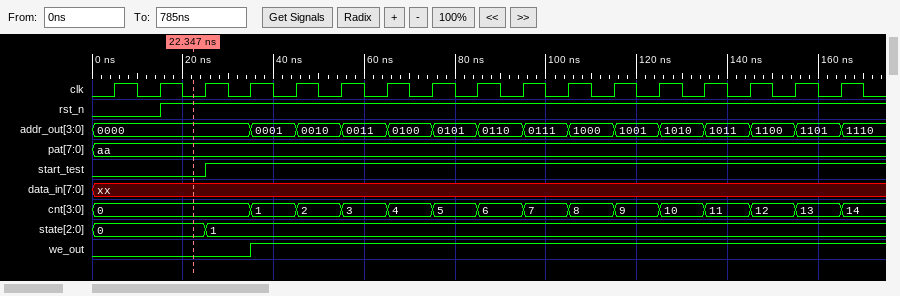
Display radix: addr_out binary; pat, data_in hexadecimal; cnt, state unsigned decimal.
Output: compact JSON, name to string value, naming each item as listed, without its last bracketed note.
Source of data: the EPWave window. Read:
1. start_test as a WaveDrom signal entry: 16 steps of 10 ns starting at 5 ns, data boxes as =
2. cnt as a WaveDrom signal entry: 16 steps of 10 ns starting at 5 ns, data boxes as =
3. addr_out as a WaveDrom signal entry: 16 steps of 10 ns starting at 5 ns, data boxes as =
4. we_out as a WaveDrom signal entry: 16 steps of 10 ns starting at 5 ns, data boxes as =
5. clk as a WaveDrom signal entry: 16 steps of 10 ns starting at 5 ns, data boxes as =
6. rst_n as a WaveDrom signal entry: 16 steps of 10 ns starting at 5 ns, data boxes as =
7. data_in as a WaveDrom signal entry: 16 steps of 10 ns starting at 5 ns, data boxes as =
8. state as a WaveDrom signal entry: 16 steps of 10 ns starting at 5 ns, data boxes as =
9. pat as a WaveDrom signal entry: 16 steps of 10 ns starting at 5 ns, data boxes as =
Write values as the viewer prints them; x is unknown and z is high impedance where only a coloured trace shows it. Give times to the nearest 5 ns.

{"start_test as a WaveDrom signal entry: 16 steps of 10 ns starting at 5 ns, data boxes as =": "{name: 'start_test', wave: '0.1.............'}", "cnt as a WaveDrom signal entry: 16 steps of 10 ns starting at 5 ns, data boxes as =": "{name: 'cnt', wave: '=..=============', data: '0 1 2 3 4 5 6 7 8 9 10 11 12 13'}", "addr_out as a WaveDrom signal entry: 16 steps of 10 ns starting at 5 ns, data boxes as =": "{name: 'addr_out', wave: '=..=============', data: '0000 0001 0010 0011 0100 0101 0110 0111 1000 1001 1010 1011 1100 1101'}", "we_out as a WaveDrom signal entry: 16 steps of 10 ns starting at 5 ns, data boxes as =": "{name: 'we_out', wave: '0..1............'}", "clk as a WaveDrom signal entry: 16 steps of 10 ns starting at 5 ns, data boxes as =": "{name: 'clk', wave: 'p...............'}", "rst_n as a WaveDrom signal entry: 16 steps of 10 ns starting at 5 ns, data boxes as =": "{name: 'rst_n', wave: '01..............'}", "data_in as a WaveDrom signal entry: 16 steps of 10 ns starting at 5 ns, data boxes as =": "{name: 'data_in', wave: 'x...............'}", "state as a WaveDrom signal entry: 16 steps of 10 ns starting at 5 ns, data boxes as =": "{name: 'state', wave: '=.=.............', data: '0 1'}", "pat as a WaveDrom signal entry: 16 steps of 10 ns starting at 5 ns, data boxes as =": "{name: 'pat', wave: '=...............', data: 'aa'}"}
